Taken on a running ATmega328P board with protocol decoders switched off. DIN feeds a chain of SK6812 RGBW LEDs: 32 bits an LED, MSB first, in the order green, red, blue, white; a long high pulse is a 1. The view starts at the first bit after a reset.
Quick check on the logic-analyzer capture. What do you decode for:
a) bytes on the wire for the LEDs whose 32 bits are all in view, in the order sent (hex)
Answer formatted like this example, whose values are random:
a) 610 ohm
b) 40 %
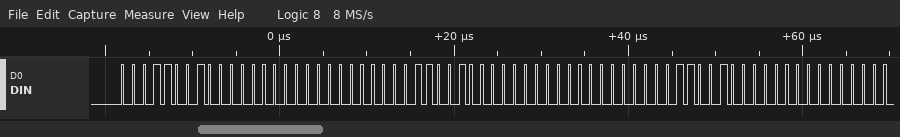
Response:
a) 19 00 00 19 00 00 19 00
